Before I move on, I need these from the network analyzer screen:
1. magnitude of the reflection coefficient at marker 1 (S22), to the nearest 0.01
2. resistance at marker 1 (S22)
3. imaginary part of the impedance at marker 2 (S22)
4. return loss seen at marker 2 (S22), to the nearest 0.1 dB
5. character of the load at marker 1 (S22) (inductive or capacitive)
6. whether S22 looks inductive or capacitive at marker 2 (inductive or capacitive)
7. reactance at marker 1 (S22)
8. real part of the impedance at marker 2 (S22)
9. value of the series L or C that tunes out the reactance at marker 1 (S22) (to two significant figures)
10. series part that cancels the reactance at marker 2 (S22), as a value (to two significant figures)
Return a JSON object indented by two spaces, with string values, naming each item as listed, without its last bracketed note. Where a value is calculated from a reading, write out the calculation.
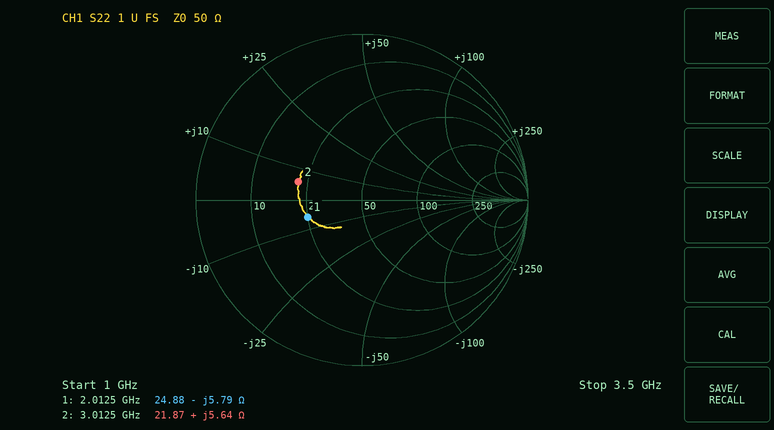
{
  "magnitude of the reflection coefficient at marker 1 (S22), to the nearest 0.01": "0.34",
  "resistance at marker 1": "24.88 Ω",
  "imaginary part of the impedance at marker 2": "+5.64 Ω",
  "return loss seen at marker 2 (S22), to the nearest 0.1 dB": "8.0 dB",
  "character of the load at marker 1 (S22)": "capacitive",
  "whether S22 looks inductive or capacitive at marker 2": "inductive",
  "reactance at marker 1": "-5.79 Ω",
  "real part of the impedance at marker 2": "21.87 Ω",
  "value of the series L or C that tunes out the reactance at marker 1 (S22)": "L = 5.79 Ω/(2π × 2.0125 GHz) ≈ 458 pH, so 460 pH to two significant figures",
  "series part that cancels the reactance at marker 2 (S22), as a value": "C = 1/(2π × 3.0125 GHz × 5.64 Ω) ≈ 9.4 pF"
}
